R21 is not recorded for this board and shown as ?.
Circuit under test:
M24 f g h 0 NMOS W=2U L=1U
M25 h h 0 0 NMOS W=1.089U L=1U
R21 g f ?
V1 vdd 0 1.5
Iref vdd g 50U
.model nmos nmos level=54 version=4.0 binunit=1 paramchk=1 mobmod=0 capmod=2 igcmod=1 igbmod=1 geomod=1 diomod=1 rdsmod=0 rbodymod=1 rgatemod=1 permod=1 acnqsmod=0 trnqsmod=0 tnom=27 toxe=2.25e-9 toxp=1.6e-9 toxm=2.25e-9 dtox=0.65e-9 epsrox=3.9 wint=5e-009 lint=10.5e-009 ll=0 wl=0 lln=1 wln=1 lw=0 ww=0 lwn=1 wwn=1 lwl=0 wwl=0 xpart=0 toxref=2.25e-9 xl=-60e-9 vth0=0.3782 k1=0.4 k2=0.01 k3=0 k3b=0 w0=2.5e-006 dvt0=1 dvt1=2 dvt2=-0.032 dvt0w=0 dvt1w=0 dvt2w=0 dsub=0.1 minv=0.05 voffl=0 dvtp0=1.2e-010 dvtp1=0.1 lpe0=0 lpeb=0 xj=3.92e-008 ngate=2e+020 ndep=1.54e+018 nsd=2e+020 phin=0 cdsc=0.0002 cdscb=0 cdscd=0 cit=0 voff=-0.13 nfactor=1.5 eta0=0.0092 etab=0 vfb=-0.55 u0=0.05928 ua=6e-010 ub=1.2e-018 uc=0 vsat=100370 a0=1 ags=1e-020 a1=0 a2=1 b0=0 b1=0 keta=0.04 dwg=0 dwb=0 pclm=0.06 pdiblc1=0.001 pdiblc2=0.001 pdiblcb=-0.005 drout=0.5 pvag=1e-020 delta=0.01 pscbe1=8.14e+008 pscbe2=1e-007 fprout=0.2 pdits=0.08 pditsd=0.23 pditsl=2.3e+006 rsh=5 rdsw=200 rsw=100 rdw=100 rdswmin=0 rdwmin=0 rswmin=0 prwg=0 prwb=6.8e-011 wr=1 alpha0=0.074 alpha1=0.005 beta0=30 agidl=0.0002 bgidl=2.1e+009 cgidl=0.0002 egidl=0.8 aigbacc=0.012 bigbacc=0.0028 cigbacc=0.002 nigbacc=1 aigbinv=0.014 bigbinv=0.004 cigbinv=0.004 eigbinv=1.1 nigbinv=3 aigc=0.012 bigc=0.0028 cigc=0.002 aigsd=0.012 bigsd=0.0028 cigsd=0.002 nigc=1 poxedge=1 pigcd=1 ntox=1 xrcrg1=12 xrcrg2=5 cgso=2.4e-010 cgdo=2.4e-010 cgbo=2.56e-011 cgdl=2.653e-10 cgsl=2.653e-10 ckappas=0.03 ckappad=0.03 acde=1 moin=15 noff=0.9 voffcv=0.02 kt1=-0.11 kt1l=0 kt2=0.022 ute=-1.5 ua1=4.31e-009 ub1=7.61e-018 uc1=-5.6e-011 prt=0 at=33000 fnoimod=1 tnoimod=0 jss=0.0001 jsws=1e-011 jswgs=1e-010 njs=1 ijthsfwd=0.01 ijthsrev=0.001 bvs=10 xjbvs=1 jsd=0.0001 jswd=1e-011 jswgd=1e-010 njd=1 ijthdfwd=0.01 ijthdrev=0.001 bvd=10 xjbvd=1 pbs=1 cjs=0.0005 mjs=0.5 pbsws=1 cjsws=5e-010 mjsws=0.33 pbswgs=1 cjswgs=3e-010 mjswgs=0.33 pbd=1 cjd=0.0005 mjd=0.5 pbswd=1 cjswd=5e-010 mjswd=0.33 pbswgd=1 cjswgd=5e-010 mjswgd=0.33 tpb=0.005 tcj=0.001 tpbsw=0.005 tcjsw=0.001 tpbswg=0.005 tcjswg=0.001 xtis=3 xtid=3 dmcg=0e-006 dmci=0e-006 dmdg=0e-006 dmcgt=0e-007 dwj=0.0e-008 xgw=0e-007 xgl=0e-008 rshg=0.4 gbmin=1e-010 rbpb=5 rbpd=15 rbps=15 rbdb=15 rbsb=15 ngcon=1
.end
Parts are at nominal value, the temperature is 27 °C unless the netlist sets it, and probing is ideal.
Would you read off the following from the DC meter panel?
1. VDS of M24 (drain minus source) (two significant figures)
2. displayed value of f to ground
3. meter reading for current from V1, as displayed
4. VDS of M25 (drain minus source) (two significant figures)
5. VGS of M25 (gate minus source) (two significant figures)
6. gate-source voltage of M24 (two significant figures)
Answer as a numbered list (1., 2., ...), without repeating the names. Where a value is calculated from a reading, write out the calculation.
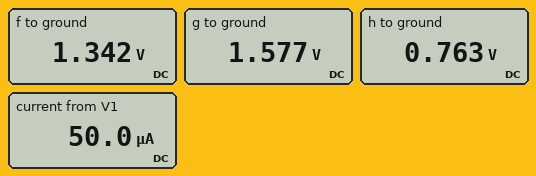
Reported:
1. 1.342 V - 763 mV = 580 mV
2. 1.342 V
3. 50.0 µA
4. 763 mV = 760 mV
5. 763 mV = 760 mV
6. 1.577 V - 763 mV = 810 mV
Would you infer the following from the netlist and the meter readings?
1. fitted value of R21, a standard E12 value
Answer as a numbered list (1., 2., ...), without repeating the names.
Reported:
1. 4.7 kΩ
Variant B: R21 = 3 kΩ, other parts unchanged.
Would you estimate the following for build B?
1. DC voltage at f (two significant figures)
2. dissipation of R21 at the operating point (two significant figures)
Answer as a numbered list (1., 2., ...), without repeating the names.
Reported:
1. 1.4 V
2. 7.5 µW
